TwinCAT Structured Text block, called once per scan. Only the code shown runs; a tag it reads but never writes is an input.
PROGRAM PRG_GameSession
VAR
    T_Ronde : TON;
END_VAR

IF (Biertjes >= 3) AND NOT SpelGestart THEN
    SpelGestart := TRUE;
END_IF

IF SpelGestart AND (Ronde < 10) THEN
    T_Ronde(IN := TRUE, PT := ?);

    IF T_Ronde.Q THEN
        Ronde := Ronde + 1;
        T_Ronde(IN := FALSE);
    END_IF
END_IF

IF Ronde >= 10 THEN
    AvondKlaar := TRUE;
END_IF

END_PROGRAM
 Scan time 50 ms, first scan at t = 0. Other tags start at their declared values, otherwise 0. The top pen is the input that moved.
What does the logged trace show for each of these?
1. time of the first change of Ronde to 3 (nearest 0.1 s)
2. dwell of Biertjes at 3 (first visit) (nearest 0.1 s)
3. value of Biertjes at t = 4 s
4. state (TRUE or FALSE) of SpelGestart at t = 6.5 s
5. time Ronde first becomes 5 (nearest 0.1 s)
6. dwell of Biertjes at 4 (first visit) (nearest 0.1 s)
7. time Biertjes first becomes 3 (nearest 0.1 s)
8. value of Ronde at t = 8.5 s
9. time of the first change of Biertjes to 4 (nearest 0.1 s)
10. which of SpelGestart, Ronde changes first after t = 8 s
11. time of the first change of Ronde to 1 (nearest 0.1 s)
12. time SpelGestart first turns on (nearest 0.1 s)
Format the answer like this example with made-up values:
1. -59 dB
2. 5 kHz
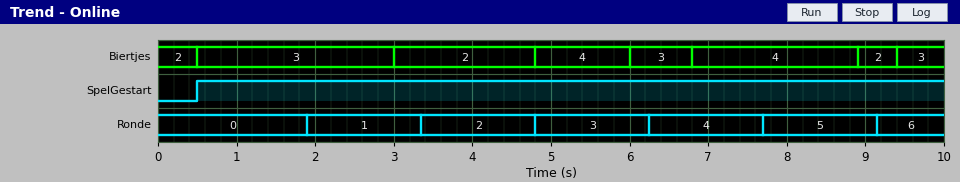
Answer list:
1. 4.8 s
2. 2.5 s
3. 2
4. TRUE
5. 7.7 s
6. 1.2 s
7. 0.5 s
8. 5
9. 4.8 s
10. Ronde
11. 1.9 s
12. 0.5 s
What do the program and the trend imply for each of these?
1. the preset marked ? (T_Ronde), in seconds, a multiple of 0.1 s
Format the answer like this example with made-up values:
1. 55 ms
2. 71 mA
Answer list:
1. 1.4 s
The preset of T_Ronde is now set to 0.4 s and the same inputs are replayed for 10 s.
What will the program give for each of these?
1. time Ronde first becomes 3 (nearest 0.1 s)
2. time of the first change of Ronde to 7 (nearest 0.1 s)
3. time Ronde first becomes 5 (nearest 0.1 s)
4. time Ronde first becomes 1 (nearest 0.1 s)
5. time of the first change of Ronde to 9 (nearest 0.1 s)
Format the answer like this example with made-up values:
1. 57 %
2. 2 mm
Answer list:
1. 1.8 s
2. 3.6 s
3. 2.7 s
4. 0.9 s
5. 4.5 s
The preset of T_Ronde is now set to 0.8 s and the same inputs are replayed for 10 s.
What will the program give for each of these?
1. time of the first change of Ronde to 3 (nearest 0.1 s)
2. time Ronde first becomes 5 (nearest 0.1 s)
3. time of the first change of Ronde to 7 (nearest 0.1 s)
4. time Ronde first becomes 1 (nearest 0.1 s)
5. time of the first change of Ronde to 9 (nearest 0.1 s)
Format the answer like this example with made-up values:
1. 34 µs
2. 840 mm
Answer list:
1. 3.0 s
2. 4.7 s
3. 6.4 s
4. 1.3 s
5. 8.1 s
